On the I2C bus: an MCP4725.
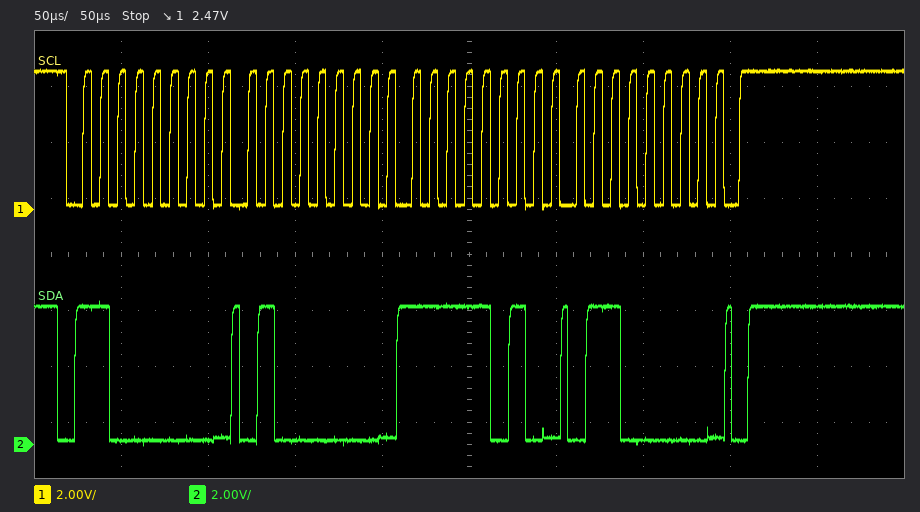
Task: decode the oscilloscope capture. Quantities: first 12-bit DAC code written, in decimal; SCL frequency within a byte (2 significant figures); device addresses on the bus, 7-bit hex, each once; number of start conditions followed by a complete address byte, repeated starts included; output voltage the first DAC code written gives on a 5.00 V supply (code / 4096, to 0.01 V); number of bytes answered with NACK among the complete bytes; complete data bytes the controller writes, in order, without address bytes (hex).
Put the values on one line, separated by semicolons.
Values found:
4006; 100 kHz; 0x60; 1; 4.89 V; 0; 40 FA 60
